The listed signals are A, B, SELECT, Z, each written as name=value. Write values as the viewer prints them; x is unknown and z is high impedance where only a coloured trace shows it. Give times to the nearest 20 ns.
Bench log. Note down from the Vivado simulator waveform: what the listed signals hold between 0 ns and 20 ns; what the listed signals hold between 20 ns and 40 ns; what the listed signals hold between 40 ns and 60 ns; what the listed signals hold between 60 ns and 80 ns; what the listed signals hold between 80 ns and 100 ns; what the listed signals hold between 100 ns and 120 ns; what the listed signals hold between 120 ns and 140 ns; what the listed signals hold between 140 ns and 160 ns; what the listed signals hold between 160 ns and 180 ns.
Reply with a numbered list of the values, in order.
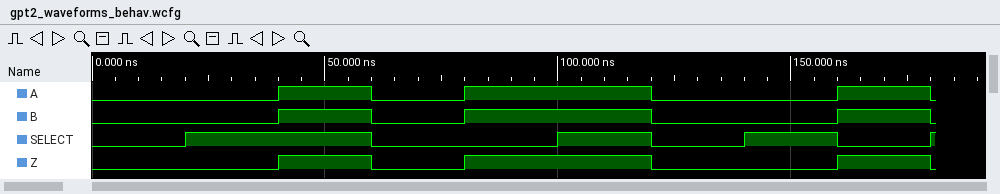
1. A=0, B=0, SELECT=0, Z=0
2. A=0, B=0, SELECT=1, Z=0
3. A=1, B=1, SELECT=1, Z=1
4. A=0, B=0, SELECT=0, Z=0
5. A=1, B=1, SELECT=0, Z=1
6. A=1, B=1, SELECT=1, Z=1
7. A=0, B=0, SELECT=0, Z=0
8. A=0, B=0, SELECT=1, Z=0
9. A=1, B=1, SELECT=0, Z=1
